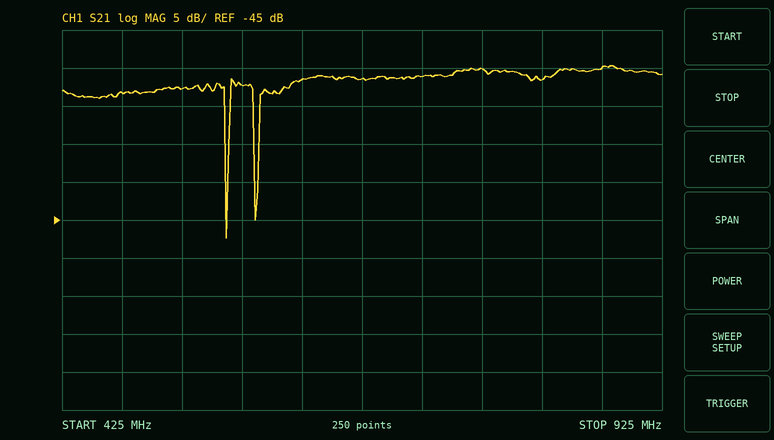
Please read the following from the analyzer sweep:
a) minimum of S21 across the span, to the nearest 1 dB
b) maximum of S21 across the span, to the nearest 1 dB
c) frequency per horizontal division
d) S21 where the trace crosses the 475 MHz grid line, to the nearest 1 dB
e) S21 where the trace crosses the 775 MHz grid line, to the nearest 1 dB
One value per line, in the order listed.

-47 dB
-25 dB
50 MHz
-28 dB
-25 dB
